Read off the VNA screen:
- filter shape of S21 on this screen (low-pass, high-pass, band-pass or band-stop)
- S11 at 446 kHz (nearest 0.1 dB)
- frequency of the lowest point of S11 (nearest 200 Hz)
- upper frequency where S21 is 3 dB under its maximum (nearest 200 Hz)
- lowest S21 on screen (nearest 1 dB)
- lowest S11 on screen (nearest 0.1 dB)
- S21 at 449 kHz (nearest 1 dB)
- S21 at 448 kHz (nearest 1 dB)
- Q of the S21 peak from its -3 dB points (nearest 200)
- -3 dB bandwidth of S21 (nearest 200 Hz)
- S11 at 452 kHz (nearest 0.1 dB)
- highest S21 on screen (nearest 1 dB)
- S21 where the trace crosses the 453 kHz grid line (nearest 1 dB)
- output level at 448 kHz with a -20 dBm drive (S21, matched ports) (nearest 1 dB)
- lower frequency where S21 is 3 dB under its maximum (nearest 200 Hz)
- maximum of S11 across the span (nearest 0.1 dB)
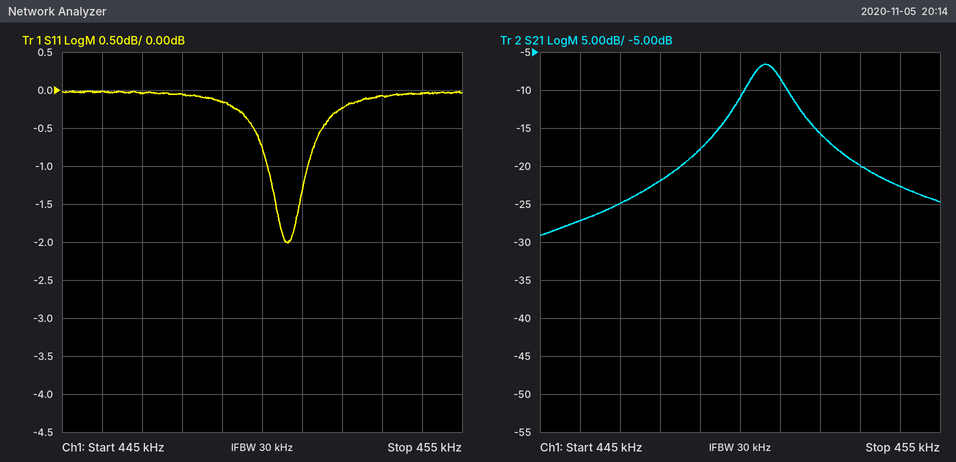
band-pass
0.0 dB
450.6 kHz
451.2 kHz
-29 dB
-2.0 dB
-18 dB
-22 dB
400
1.0 kHz
-0.2 dB
-7 dB
-20 dB
-42 dBm
450.2 kHz
0.0 dB
